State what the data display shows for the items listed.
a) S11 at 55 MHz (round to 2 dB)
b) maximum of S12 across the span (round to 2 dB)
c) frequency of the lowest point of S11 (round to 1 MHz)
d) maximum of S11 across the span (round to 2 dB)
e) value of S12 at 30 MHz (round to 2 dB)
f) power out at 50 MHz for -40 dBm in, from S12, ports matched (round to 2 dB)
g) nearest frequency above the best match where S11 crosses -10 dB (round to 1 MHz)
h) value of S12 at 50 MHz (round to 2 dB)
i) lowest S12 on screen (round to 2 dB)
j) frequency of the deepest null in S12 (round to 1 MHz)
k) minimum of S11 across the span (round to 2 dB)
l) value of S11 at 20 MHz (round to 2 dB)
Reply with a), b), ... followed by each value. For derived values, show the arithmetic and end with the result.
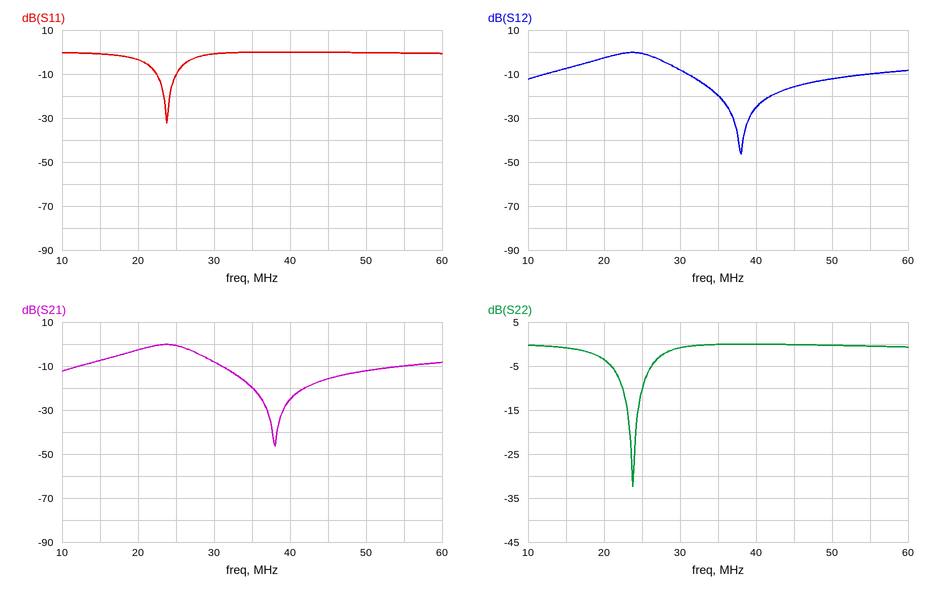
a) 0 dB
b) 0 dB
c) 24 MHz
d) 0 dB
e) -8 dB
f) -40 dBm + (-12 dB) = -52 dBm
g) 25 MHz
h) -12 dB
i) -46 dB
j) 38 MHz
k) -32 dB
l) -4 dB
